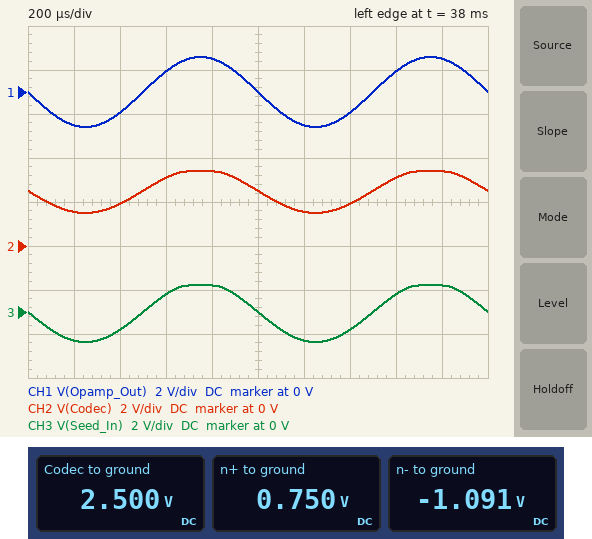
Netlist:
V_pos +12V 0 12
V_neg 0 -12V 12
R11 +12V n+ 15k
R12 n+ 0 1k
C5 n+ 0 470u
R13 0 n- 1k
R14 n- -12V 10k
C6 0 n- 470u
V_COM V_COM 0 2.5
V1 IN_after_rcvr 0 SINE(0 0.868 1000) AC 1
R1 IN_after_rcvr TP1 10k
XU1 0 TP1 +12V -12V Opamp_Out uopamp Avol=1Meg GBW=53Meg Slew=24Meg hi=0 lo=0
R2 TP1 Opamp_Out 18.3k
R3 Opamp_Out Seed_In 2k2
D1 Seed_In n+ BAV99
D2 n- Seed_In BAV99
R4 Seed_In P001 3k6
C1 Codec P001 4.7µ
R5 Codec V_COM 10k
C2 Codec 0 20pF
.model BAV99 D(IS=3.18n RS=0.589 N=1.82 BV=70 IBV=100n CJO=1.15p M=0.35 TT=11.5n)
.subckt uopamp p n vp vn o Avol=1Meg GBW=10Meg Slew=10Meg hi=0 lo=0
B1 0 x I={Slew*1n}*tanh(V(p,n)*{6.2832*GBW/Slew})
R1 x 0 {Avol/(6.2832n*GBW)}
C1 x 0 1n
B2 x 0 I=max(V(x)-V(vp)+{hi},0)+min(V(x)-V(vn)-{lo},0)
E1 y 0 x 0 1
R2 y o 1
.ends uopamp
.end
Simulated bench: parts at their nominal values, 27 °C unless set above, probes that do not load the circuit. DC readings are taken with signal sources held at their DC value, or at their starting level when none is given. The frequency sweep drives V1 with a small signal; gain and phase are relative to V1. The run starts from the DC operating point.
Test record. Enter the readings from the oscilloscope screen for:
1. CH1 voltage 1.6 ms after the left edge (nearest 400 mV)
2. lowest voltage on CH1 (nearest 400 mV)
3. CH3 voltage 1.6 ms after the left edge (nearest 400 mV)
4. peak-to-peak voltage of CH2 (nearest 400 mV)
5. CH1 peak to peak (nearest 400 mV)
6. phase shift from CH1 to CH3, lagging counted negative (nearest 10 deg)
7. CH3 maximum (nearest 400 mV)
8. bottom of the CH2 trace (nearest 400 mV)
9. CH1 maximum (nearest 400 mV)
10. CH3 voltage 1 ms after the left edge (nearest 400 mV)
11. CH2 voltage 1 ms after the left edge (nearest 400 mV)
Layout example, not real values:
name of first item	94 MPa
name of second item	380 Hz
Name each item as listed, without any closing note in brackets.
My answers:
CH1 voltage 1.6 ms after the left edge	800 mV
lowest voltage on CH1	-1.6 V
CH3 voltage 1.6 ms after the left edge	800 mV
peak-to-peak voltage of CH2	2.0 V
CH1 peak to peak	3.2 V
phase shift from CH1 to CH3, lagging counted negative	0 deg
CH3 maximum	1.2 V
bottom of the CH2 trace	1.6 V
CH1 maximum	1.6 V
CH3 voltage 1 ms after the left edge	0 V
CH2 voltage 1 ms after the left edge	2.4 V
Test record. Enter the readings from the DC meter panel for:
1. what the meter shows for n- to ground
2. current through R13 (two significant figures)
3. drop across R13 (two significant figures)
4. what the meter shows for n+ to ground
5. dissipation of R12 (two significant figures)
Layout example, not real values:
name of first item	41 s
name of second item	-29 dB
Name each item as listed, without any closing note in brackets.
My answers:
what the meter shows for n- to ground	-1.091 V
current through R13	1.1 mA
drop across R13	1.1 V
what the meter shows for n+ to ground	0.750 V
dissipation of R12	560 µW
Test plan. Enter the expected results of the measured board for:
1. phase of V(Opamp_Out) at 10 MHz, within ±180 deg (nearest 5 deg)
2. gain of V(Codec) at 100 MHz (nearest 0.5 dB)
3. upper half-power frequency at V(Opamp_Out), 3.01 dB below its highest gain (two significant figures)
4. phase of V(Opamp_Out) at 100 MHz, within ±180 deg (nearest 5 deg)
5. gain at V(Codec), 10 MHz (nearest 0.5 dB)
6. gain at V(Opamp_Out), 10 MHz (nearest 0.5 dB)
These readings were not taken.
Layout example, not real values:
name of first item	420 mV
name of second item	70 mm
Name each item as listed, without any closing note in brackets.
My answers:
phase of V(Opamp_Out) at 10 MHz, within ±180 deg	150 deg
gain of V(Codec) at 100 MHz	-52.0 dB
upper half-power frequency at V(Opamp_Out), 3.01 dB below its highest gain	19 MHz
phase of V(Opamp_Out) at 100 MHz, within ±180 deg	100 deg
gain at V(Codec), 10 MHz	-13.5 dB
gain at V(Opamp_Out), 10 MHz	4.0 dB
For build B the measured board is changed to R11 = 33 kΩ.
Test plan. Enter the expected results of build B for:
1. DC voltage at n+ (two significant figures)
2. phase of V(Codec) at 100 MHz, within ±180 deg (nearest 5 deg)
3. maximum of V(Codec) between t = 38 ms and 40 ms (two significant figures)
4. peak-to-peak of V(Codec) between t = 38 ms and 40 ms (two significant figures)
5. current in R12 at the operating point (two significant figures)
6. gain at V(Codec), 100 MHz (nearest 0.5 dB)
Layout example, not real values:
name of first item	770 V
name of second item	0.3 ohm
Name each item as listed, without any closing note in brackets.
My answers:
DC voltage at n+	350 mV
phase of V(Codec) at 100 MHz, within ±180 deg	-45 deg
maximum of V(Codec) between t = 38 ms and 40 ms	3.2 V
peak-to-peak of V(Codec) between t = 38 ms and 40 ms	1.7 V
current in R12 at the operating point	350 µA
gain at V(Codec), 100 MHz	-52.5 dB
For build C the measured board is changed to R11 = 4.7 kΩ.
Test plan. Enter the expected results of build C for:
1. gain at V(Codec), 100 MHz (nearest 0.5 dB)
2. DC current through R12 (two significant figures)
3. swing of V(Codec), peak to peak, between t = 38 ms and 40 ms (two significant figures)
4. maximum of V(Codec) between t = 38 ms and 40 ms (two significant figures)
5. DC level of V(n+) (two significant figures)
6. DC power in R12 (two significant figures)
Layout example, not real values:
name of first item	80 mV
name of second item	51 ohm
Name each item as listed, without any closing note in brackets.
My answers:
gain at V(Codec), 100 MHz	-51.5 dB
DC current through R12	2.1 mA
swing of V(Codec), peak to peak, between t = 38 ms and 40 ms	2.0 V
maximum of V(Codec) between t = 38 ms and 40 ms	3.5 V
DC level of V(n+)	2.1 V
DC power in R12	4.4 mW
